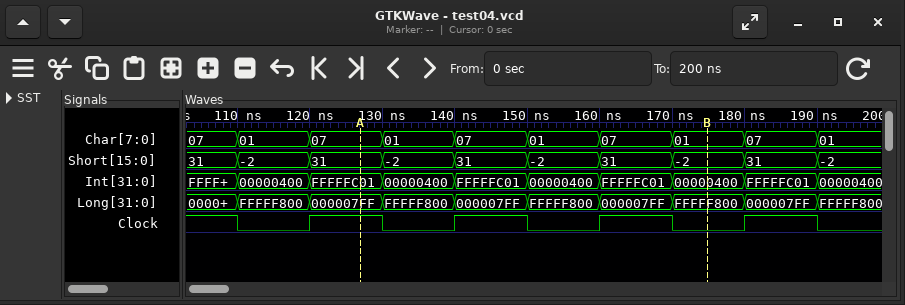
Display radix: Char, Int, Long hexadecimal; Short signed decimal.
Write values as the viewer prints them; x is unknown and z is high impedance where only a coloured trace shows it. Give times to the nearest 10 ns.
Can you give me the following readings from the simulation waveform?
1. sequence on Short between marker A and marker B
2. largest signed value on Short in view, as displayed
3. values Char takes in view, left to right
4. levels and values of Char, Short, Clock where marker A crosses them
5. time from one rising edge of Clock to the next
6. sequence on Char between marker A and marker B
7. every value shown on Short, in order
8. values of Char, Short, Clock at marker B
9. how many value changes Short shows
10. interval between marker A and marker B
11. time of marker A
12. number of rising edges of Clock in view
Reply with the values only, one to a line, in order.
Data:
31, -2, 31, -2, 31, -2
31
07, 01, 07, 01, 07, 01, 07, 01, 07, 01
Char=07, Short=31, Clock=1
20 ns
07, 01, 07, 01, 07, 01
31, -2, 31, -2, 31, -2, 31, -2, 31, -2
Char=01, Short=-2, Clock=0
9
50 ns
130 ns
4
